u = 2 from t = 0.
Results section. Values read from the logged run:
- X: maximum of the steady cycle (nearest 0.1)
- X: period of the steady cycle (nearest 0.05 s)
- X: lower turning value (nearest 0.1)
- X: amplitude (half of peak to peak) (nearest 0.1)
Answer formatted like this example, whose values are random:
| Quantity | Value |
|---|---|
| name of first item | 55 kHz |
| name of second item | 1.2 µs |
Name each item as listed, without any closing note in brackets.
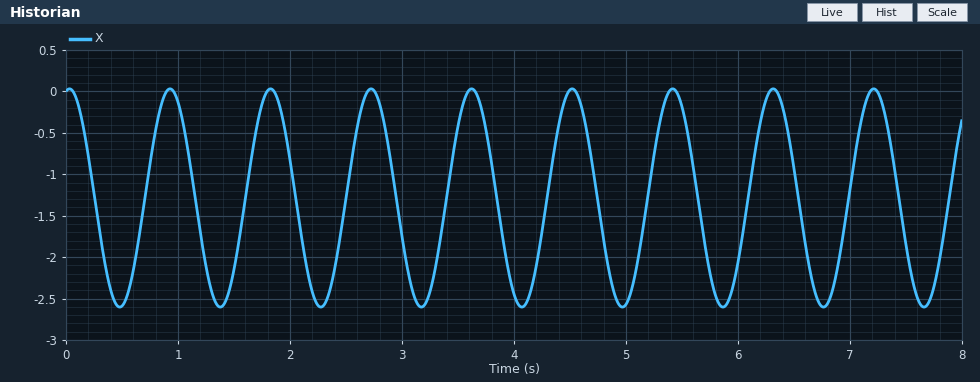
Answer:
| Quantity | Value |
|---|---|
| X: maximum of the steady cycle | 0.0 |
| X: period of the steady cycle | 0.90 s |
| X: lower turning value | -2.6 |
| X: amplitude (half of peak to peak) | 1.3 |
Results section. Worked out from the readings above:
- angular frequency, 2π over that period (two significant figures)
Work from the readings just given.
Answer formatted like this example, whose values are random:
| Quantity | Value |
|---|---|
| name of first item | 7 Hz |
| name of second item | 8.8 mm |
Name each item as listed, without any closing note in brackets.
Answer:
| Quantity | Value |
|---|---|
| angular frequency, 2π over that period | 7.0 rad/s |
